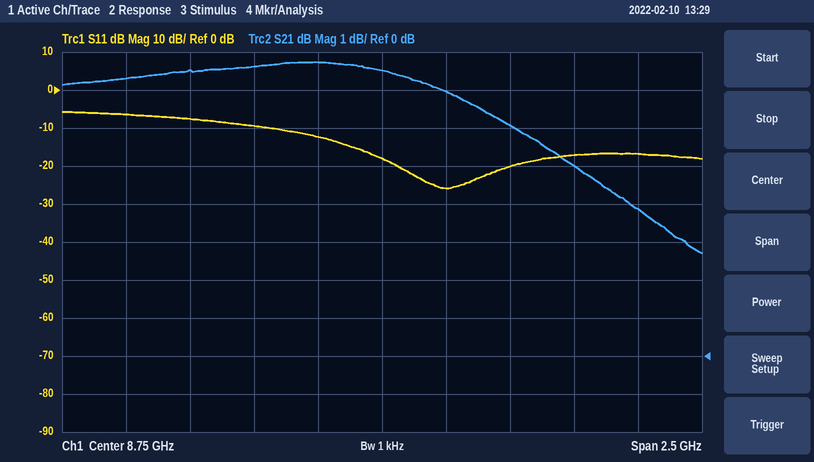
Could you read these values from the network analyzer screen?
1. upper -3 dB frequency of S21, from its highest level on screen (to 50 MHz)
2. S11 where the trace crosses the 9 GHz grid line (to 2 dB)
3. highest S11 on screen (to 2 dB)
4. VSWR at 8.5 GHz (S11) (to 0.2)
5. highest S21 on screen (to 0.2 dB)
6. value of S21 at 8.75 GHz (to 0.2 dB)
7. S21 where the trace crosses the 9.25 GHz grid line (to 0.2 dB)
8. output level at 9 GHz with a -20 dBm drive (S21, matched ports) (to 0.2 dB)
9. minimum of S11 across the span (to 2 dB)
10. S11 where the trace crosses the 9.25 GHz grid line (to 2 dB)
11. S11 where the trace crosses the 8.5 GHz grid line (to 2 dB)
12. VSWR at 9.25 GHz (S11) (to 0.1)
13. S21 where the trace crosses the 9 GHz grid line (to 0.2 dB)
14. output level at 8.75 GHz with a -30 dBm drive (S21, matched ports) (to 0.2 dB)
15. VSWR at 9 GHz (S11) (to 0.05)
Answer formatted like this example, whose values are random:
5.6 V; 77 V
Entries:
9.55 GHz; -26 dB; -6 dB; 1.6; 7.8 dB; 7.6 dB; 6.0 dB; -13.0 dBm; -26 dB; -20 dB; -12 dB; 1.2; 7.0 dB; -22.4 dBm; 1.10
